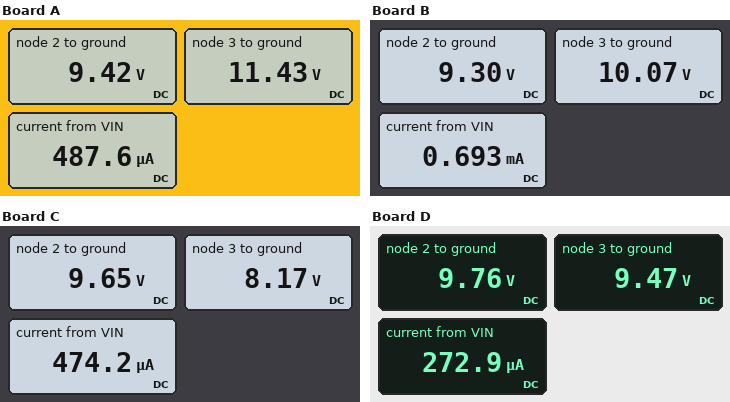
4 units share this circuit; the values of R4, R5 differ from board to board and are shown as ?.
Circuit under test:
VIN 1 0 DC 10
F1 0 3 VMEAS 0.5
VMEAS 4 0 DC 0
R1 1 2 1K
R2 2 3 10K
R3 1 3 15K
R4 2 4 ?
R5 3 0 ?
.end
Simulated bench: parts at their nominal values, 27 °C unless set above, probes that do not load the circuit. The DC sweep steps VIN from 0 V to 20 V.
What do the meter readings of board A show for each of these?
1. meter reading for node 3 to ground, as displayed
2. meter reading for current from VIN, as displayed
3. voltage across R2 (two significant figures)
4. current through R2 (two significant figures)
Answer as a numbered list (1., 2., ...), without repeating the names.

1. 11.43 V
2. 487.6 µA
3. 2.0 V
4. 200 µA
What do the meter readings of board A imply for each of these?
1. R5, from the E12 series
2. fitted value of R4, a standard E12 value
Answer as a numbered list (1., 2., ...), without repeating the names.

1. 120 kΩ
2. 12 kΩ
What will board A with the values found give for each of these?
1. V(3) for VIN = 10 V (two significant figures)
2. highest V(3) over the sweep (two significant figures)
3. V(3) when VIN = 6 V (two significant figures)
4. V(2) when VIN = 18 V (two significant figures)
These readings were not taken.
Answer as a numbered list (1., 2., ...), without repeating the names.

1. 11 V
2. 23 V
3. 6.9 V
4. 17 V
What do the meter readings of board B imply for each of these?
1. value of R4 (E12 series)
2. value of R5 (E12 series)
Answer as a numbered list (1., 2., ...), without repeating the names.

1. 12 kΩ
2. 33 kΩ
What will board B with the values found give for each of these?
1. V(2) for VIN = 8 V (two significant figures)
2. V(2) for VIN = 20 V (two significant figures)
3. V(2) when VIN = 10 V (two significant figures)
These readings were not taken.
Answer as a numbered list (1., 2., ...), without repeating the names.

1. 7.4 V
2. 19 V
3. 9.3 V
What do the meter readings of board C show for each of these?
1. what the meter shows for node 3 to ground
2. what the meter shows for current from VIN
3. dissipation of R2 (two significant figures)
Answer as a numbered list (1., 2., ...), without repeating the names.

1. 8.17 V
2. 474.2 µA
3. 220 µW
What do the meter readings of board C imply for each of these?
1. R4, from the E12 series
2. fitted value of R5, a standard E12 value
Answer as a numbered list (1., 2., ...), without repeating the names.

1. 47 kΩ
2. 22 kΩ
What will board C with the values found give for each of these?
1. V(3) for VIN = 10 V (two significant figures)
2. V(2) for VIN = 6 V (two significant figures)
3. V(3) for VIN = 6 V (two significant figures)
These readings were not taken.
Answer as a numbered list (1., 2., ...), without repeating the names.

1. 8.2 V
2. 5.8 V
3. 4.9 V
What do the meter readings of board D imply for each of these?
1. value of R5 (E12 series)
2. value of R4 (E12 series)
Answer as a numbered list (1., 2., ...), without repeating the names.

1. 56 kΩ
2. 47 kΩ
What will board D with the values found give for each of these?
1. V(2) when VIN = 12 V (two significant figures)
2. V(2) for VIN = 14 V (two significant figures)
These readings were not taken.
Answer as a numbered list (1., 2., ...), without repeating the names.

1. 12 V
2. 14 V
